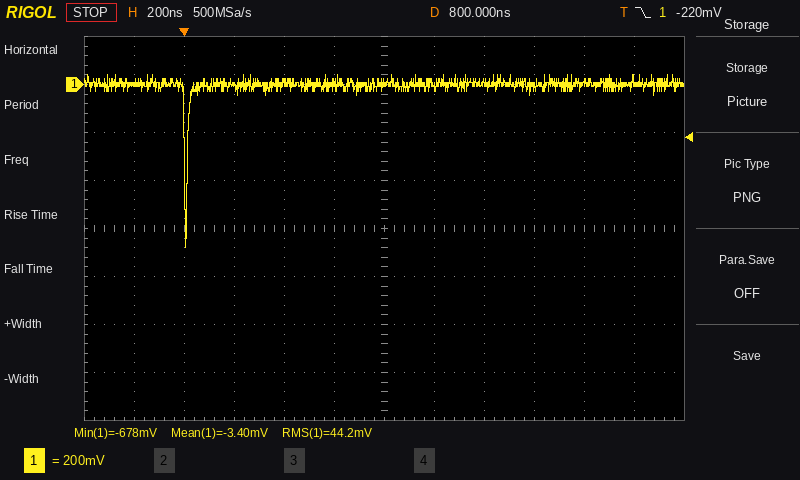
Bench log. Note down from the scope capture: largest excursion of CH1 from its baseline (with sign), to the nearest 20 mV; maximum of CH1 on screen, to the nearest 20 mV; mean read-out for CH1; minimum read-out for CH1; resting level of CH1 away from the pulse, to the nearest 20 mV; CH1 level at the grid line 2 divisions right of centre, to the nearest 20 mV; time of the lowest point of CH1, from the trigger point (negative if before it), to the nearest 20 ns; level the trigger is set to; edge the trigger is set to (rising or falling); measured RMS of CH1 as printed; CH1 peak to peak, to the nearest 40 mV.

-680 mV
40 mV
-3.40 mV
-678 mV
0 mV
0 mV
0 ns
-220 mV
falling
44.2 mV
720 mV
